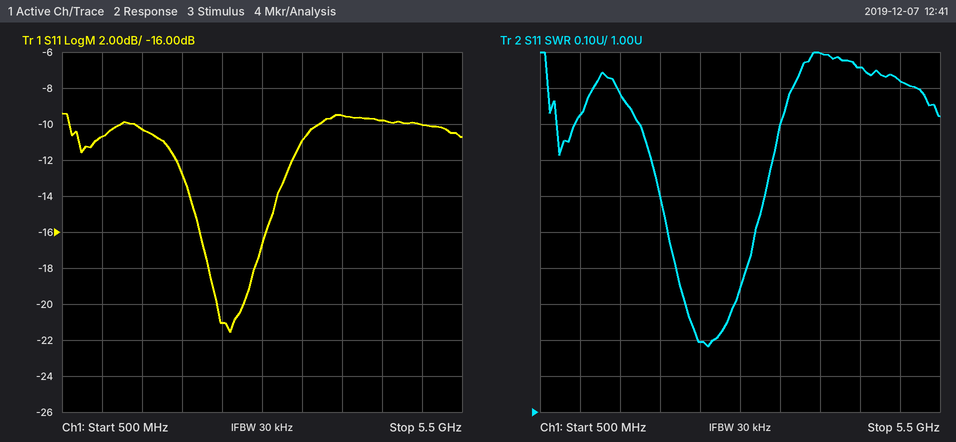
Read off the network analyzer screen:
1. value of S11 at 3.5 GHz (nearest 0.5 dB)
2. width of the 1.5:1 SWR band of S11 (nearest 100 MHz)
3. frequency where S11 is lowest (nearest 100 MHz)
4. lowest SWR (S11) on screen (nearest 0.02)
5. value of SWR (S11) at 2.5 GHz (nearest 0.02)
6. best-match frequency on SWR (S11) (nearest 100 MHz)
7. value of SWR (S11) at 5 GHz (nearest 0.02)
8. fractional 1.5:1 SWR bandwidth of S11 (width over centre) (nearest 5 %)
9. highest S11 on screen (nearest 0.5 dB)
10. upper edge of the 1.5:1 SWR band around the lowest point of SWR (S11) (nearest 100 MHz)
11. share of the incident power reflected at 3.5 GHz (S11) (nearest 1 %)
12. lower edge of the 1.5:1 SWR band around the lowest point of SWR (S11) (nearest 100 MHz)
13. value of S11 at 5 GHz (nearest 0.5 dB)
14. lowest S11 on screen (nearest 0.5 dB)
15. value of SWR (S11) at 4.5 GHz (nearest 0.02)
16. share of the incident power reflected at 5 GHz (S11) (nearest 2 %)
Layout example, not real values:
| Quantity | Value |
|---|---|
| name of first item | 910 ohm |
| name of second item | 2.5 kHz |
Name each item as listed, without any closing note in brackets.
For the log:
| Quantity | Value |
|---|---|
| value of S11 at 3.5 GHz | -11.0 dB |
| width of the 1.5:1 SWR band of S11 | 1.1 GHz |
| frequency where S11 is lowest | 2.6 GHz |
| lowest SWR (S11) on screen | 1.18 |
| value of SWR (S11) at 2.5 GHz | 1.20 |
| best-match frequency on SWR (S11) | 2.6 GHz |
| value of SWR (S11) at 5 GHz | 1.92 |
| fractional 1.5:1 SWR bandwidth of S11 (width over centre) | 40 % |
| highest S11 on screen | -9.5 dB |
| upper edge of the 1.5:1 SWR band around the lowest point of SWR (S11) | 3.2 GHz |
| share of the incident power reflected at 3.5 GHz (S11) | 8 % |
| lower edge of the 1.5:1 SWR band around the lowest point of SWR (S11) | 2.1 GHz |
| value of S11 at 5 GHz | -10.0 dB |
| lowest S11 on screen | -21.5 dB |
| value of SWR (S11) at 4.5 GHz | 1.96 |
| share of the incident power reflected at 5 GHz (S11) | 10 % |
